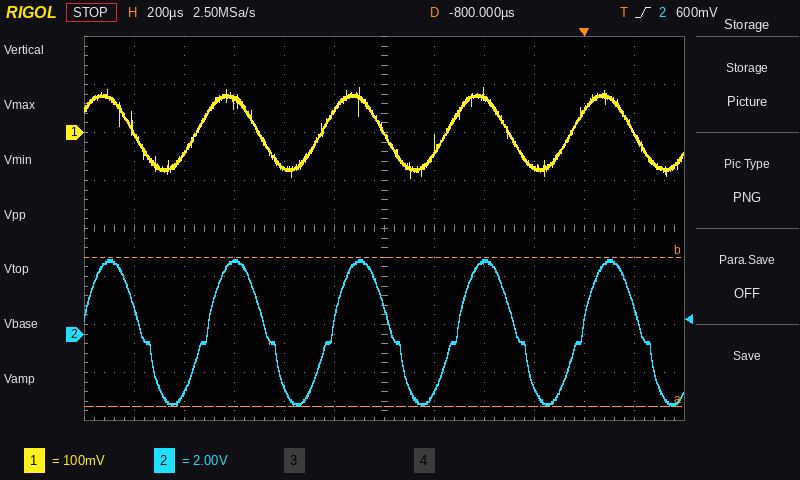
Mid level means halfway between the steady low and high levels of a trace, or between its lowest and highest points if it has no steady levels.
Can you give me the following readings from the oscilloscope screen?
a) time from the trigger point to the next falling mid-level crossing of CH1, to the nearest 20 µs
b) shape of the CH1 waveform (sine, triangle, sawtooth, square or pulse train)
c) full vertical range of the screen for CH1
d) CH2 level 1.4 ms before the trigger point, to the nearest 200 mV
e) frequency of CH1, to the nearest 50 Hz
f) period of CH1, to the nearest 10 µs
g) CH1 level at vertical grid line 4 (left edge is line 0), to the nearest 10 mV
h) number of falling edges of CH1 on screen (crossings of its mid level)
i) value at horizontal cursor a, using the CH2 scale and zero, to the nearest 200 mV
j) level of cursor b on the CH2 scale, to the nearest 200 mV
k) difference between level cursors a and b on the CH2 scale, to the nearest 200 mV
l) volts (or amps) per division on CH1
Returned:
200 µs
sine
800 mV
3.0 V
2.00 kHz
500 µs
-70 mV
5
-3.0 V
3.2 V
6.2 V
100 mV
